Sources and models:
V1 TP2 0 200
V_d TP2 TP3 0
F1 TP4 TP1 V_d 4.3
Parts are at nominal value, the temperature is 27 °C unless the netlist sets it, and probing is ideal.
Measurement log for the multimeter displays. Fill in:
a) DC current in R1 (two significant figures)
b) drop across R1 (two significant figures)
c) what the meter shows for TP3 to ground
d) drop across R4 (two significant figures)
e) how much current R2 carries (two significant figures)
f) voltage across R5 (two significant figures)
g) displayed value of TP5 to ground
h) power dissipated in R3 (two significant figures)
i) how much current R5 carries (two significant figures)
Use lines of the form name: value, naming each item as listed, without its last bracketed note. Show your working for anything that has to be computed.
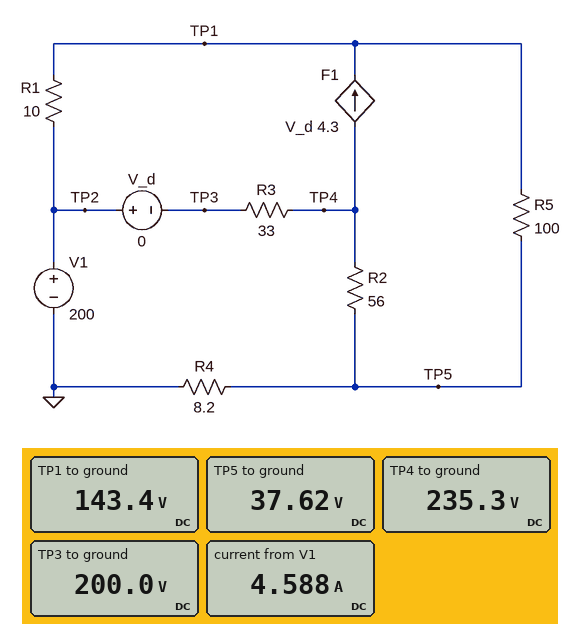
DC current in R1: (200 V - 143.4 V) / 10 Ω = 5.7 A
drop across R1: 200 V - 143.4 V = 57 V
what the meter shows for TP3 to ground: 200.0 V
drop across R4: 37.62 V = 38 V
how much current R2 carries: (235.3 V - 37.62 V) / 56 Ω = 3.5 A
voltage across R5: 143.4 V - 37.62 V = 110 V
displayed value of TP5 to ground: 37.62 V
power dissipated in R3: (235.3 V - 200 V)^2 / 33 Ω = 38 W
how much current R5 carries: (143.4 V - 37.62 V) / 100 Ω = 1.1 A
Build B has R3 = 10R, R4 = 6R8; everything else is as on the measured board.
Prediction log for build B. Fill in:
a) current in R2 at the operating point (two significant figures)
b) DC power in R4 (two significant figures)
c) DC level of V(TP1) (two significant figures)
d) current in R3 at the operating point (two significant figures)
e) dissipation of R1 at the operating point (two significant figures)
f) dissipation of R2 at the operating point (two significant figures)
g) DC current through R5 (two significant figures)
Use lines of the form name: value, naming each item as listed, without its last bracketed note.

current in R2 at the operating point: 3.2 A
DC power in R4: 130 W
DC level of V(TP1): 150 V
current in R3 at the operating point: 970 mA
dissipation of R1 at the operating point: 290 W
dissipation of R2 at the operating point: 580 W
DC current through R5: 1.2 A
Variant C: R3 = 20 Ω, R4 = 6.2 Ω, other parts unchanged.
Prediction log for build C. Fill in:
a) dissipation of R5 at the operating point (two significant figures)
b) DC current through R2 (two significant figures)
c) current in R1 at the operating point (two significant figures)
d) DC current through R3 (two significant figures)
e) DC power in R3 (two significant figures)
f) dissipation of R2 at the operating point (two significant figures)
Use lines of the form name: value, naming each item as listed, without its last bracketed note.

dissipation of R5 at the operating point: 130 W
DC current through R2: 3.4 A
current in R1 at the operating point: 5.6 A
DC current through R3: 1.0 A
DC power in R3: 22 W
dissipation of R2 at the operating point: 660 W
